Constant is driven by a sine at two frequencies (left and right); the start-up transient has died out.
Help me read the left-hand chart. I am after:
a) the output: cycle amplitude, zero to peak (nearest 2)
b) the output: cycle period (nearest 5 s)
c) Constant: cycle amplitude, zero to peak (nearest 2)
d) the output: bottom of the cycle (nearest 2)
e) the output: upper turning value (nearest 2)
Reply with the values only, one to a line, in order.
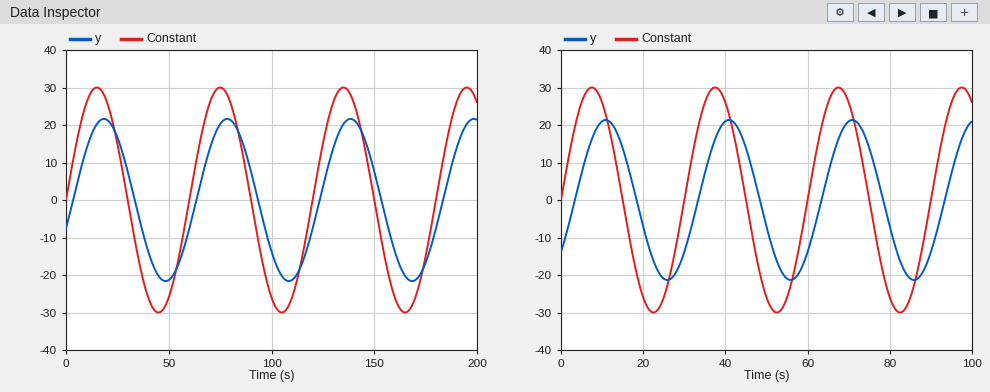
22
60 s
30
-22
22
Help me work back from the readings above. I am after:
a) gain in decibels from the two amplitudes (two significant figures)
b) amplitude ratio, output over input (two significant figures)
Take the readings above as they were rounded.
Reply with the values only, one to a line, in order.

-2.7 dB
0.73
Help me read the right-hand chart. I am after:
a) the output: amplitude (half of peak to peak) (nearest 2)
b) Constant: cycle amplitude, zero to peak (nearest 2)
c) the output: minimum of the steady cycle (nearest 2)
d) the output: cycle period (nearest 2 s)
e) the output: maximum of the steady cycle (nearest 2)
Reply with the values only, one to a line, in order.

22
30
-22
30 s
22
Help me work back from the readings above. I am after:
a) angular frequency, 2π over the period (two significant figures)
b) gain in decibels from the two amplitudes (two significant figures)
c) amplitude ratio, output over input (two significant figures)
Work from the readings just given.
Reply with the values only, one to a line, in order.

0.21 rad/s
-2.7 dB
0.73
